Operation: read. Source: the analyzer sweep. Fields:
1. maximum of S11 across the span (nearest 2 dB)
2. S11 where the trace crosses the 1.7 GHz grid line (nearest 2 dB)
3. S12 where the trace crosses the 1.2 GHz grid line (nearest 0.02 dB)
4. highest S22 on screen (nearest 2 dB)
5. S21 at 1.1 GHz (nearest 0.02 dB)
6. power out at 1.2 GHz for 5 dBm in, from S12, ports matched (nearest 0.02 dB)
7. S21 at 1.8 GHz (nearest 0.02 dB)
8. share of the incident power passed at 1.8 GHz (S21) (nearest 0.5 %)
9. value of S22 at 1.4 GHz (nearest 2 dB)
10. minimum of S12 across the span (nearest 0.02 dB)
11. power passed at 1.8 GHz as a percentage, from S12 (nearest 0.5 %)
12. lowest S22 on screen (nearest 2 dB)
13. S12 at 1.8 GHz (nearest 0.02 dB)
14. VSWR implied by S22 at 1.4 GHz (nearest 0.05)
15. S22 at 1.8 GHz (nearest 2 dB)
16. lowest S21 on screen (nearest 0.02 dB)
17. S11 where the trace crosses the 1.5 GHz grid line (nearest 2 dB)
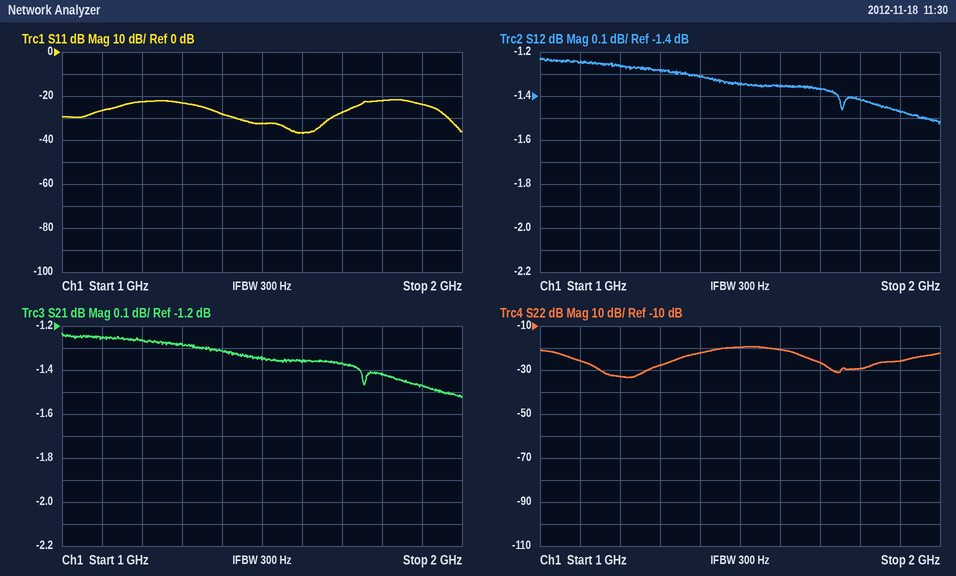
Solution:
-22 dB
-28 dB
-1.26 dB
-20 dB
-1.26 dB
3.74 dBm
-1.42 dB
72.0 %
-22 dB
-1.52 dB
72.0 %
-34 dB
-1.42 dB
1.15
-30 dB
-1.52 dB
-32 dB
